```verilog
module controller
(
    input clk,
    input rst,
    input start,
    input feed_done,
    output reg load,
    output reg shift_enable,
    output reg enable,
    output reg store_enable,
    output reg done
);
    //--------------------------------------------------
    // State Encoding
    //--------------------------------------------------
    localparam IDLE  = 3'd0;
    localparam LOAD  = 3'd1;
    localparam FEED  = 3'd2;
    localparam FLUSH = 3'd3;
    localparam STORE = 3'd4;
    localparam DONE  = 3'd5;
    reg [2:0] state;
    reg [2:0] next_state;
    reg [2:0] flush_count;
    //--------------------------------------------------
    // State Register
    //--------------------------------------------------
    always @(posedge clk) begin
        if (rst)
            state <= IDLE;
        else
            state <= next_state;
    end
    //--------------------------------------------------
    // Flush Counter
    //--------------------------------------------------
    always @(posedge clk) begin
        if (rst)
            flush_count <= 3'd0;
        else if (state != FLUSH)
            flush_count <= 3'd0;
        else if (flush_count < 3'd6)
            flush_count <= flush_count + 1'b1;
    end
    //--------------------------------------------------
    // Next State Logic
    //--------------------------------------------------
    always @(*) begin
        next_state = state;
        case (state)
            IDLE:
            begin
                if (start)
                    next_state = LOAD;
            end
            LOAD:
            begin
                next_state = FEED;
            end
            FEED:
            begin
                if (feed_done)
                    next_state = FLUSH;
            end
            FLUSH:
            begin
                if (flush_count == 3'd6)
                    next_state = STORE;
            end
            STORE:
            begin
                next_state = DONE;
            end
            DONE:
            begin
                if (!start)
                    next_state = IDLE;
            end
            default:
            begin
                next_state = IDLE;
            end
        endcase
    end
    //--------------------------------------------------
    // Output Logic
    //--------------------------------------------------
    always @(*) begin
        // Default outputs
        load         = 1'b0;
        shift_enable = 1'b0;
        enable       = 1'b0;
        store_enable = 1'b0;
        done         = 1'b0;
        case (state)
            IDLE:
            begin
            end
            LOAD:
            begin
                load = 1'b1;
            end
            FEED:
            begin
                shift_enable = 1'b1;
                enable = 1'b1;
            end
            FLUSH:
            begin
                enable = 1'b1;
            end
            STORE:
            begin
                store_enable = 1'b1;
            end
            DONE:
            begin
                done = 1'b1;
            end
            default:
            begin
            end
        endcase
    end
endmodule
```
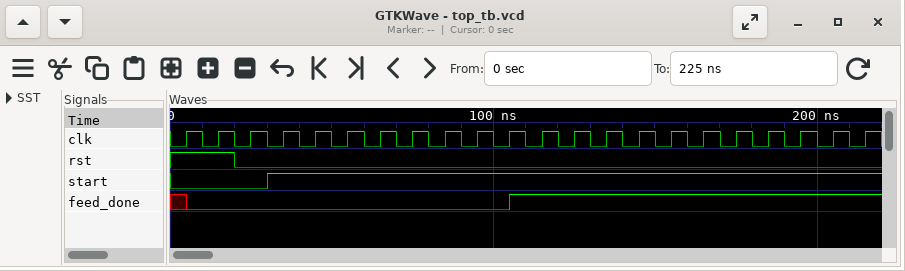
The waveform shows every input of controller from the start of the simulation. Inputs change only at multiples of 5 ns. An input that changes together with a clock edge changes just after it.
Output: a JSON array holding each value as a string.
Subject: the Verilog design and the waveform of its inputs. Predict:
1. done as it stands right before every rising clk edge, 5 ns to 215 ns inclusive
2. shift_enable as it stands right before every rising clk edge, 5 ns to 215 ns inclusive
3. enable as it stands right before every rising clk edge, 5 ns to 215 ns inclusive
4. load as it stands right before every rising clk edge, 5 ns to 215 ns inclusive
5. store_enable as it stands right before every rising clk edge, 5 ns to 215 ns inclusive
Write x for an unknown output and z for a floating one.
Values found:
["x 0 0 0 0 0 0 0 0 0 0 0 0 0 0 0 0 0 0 0 1 1", "x 0 0 0 0 1 1 1 1 1 1 1 0 0 0 0 0 0 0 0 0 0", "x 0 0 0 0 1 1 1 1 1 1 1 1 1 1 1 1 1 1 0 0 0", "x 0 0 0 1 0 0 0 0 0 0 0 0 0 0 0 0 0 0 0 0 0", "x 0 0 0 0 0 0 0 0 0 0 0 0 0 0 0 0 0 0 1 0 0"]
